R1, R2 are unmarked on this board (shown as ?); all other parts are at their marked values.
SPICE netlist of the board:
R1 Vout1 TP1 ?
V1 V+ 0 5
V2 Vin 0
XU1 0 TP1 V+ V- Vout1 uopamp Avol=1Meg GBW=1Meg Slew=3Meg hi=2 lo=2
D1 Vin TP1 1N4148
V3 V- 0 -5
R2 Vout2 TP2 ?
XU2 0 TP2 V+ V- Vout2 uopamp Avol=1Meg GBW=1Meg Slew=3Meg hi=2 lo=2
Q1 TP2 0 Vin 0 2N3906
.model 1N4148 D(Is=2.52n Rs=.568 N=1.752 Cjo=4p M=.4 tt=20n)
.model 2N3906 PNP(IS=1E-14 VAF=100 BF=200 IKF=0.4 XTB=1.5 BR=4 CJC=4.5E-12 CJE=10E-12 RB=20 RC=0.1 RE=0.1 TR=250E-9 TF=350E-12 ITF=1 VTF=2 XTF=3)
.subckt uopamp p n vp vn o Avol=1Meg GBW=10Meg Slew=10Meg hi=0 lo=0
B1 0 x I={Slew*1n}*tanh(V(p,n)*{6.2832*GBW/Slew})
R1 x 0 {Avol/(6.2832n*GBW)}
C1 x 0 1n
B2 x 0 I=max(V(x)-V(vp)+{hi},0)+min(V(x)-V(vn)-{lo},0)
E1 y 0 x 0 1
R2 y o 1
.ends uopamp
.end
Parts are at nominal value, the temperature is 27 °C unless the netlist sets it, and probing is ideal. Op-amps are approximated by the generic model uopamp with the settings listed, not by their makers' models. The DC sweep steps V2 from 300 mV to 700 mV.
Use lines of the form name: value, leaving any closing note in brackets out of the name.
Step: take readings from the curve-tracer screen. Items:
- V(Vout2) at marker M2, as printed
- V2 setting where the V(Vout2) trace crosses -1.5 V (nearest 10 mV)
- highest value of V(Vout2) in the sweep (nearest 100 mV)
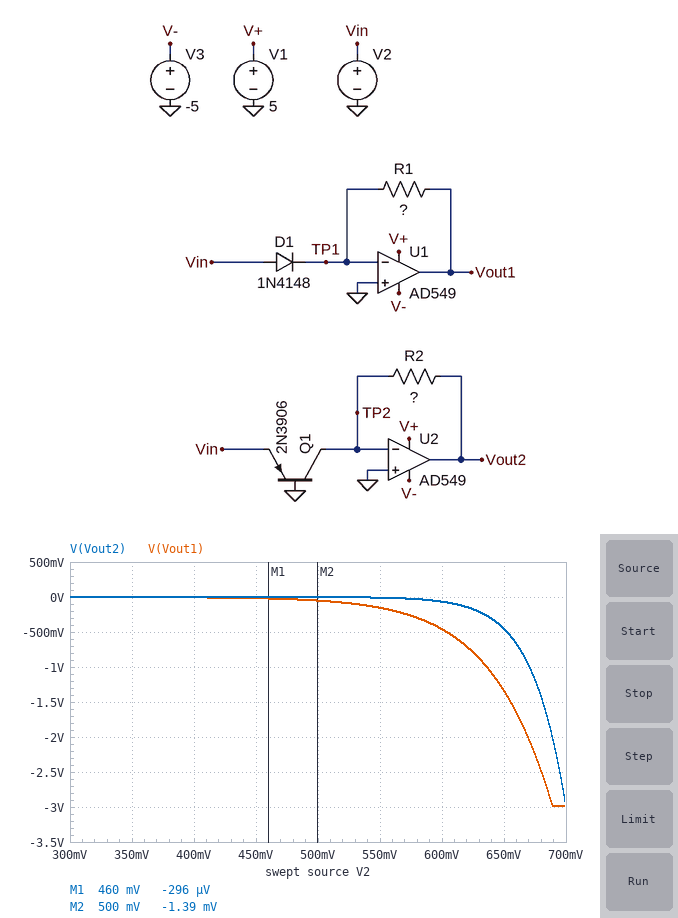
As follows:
V(Vout2) at marker M2, as printed: -1.39 mV
V2 setting where the V(Vout2) trace crosses -1.5 V: 680 mV
highest value of V(Vout2) in the sweep: 0 V
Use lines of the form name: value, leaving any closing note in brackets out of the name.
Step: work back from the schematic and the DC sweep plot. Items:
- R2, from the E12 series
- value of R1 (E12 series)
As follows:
R2, from the E12 series: 560 Ω
value of R1: 330 Ω
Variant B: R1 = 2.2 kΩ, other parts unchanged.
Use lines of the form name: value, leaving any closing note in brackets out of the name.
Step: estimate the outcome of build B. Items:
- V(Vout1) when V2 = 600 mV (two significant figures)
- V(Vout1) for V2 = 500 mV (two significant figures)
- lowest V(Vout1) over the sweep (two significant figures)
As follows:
V(Vout1) when V2 = 600 mV: -3.0 V
V(Vout1) for V2 = 500 mV: -340 mV
lowest V(Vout1) over the sweep: -3.0 V
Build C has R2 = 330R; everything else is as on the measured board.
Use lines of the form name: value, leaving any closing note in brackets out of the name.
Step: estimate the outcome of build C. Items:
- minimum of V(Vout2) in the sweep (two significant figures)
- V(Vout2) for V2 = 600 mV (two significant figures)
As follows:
minimum of V(Vout2) in the sweep: -1.8 V
V(Vout2) for V2 = 600 mV: -39 mV
